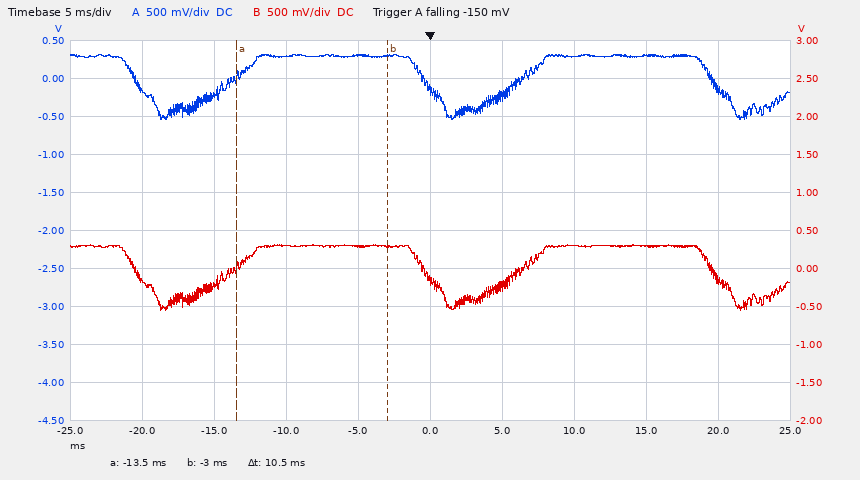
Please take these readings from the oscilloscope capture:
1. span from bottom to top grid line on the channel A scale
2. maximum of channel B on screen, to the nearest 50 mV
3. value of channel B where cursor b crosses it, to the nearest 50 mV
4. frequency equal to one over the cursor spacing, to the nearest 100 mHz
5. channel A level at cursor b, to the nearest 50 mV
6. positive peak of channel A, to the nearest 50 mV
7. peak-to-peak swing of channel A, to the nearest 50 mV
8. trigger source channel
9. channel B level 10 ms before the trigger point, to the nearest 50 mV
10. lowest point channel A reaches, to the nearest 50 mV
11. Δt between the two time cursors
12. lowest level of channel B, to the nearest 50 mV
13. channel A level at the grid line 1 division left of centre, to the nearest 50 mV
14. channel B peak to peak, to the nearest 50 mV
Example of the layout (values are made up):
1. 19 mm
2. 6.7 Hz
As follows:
1. 5 V
2. 300 mV
3. 300 mV
4. 95.2 Hz
5. 300 mV
6. 300 mV
7. 850 mV
8. channel A
9. 300 mV
10. -550 mV
11. 10.5 ms
12. -550 mV
13. 300 mV
14. 850 mV
